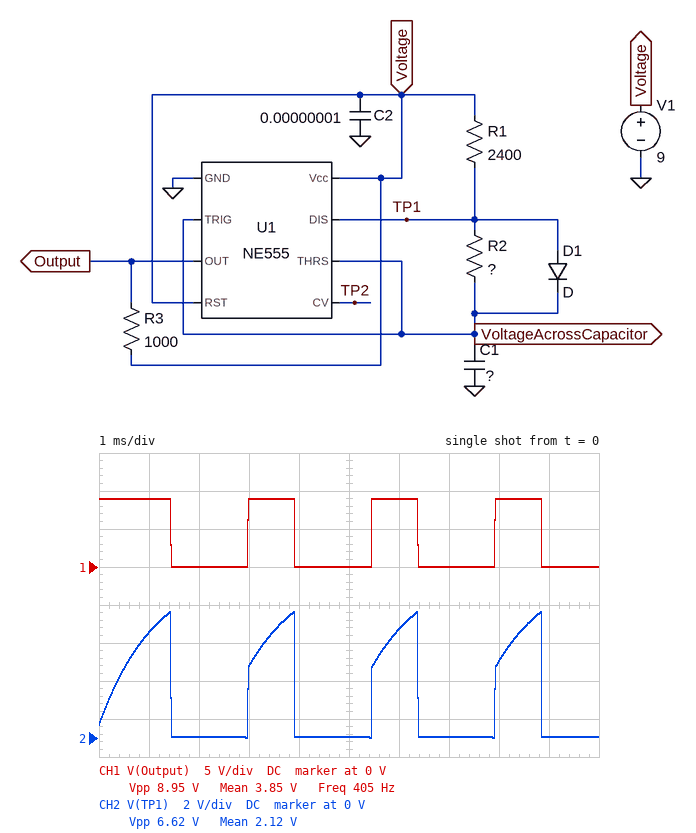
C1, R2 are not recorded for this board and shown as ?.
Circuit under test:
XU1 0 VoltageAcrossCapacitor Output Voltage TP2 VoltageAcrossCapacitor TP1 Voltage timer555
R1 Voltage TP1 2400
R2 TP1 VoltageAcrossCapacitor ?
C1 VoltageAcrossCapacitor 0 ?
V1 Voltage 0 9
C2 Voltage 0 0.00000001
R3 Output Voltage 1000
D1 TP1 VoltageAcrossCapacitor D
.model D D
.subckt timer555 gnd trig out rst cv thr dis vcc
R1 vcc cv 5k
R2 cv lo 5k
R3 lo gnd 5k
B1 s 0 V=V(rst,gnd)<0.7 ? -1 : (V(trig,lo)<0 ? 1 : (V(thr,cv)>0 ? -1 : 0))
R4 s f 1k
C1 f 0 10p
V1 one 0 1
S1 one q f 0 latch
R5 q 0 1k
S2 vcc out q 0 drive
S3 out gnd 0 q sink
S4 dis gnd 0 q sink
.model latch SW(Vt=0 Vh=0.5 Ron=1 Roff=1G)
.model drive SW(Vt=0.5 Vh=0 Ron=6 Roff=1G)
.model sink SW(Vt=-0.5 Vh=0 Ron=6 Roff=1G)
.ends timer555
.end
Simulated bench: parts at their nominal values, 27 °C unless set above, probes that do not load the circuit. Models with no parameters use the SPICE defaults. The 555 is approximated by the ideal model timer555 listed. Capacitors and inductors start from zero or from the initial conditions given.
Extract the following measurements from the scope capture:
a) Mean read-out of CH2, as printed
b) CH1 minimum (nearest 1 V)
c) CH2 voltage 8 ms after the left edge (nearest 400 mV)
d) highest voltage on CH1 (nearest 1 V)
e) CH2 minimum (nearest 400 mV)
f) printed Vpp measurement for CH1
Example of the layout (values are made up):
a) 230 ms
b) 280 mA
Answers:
a) 2.12 V
b) 0 V
c) 4.0 V
d) 9 V
e) 0 V
f) 8.95 V
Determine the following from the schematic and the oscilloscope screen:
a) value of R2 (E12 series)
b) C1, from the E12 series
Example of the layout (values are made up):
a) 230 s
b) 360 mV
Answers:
a) 4.7 kΩ
b) 470 nF
